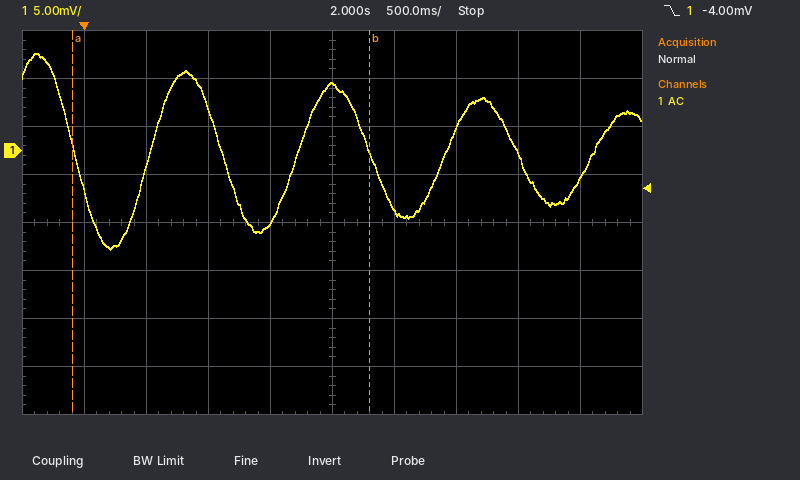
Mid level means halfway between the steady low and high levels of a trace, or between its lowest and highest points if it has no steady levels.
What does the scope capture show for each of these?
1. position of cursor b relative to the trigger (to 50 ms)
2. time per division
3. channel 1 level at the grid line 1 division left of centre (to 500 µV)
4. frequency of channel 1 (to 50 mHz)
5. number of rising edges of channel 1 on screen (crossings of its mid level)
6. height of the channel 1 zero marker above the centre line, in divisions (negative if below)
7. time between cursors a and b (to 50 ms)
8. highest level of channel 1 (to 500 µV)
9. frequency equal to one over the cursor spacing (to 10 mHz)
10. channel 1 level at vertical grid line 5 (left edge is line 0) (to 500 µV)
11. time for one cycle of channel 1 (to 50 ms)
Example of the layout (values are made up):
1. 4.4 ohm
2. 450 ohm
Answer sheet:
1. +2.30 s
2. 500 ms
3. -7.5 mV
4. 850 mHz
5. 4
6. +1.5 div
7. 2.40 s
8. 10.0 mV
9. 420 mHz
10. 7.0 mV
11. 1.20 s
